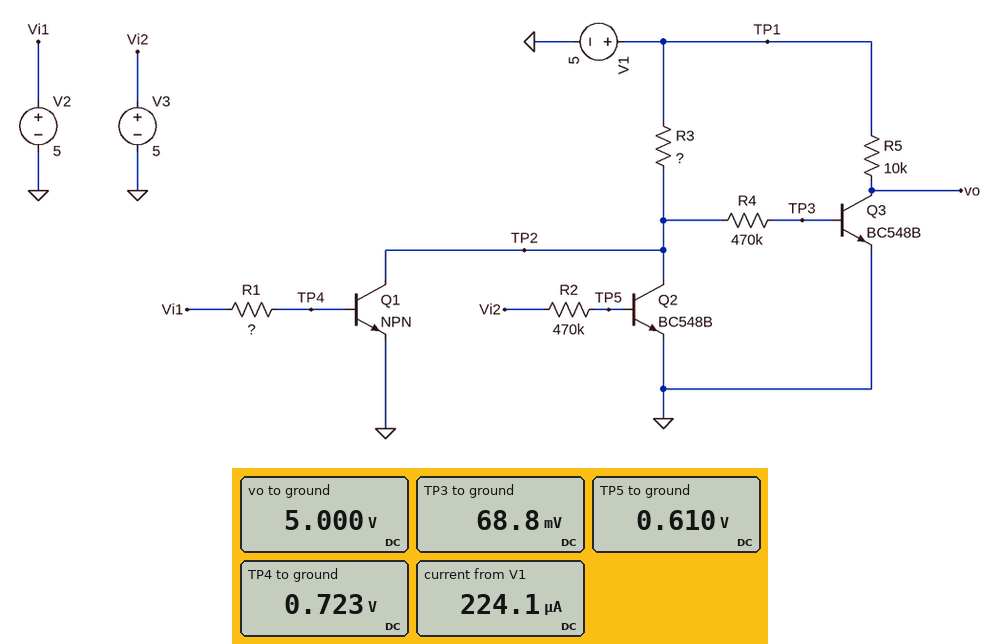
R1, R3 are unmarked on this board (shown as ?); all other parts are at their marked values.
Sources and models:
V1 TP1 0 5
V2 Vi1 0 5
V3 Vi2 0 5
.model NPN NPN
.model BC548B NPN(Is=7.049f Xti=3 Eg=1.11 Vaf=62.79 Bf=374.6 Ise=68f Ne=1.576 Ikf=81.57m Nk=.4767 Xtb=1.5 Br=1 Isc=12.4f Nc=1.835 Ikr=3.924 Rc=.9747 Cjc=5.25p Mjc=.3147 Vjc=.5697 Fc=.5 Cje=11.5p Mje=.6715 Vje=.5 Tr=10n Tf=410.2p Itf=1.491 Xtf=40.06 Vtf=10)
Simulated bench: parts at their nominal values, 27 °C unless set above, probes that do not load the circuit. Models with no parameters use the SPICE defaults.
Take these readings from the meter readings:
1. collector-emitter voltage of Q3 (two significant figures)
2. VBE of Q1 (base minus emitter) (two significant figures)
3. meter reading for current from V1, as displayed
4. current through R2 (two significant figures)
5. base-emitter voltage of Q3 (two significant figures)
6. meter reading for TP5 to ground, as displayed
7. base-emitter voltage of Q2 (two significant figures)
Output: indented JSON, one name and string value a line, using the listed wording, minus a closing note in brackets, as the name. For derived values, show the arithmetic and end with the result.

{
  "collector-emitter voltage of Q3": "5 V = 5.0 V",
  "VBE of Q1 (base minus emitter)": "723 mV = 720 mV",
  "meter reading for current from V1, as displayed": "224.1 µA",
  "current through R2": "(5 V - 610 mV) / 470 kΩ = 9.3 µA",
  "base-emitter voltage of Q3": "68.8 mV = 69 mV",
  "meter reading for TP5 to ground, as displayed": "0.610 V",
  "base-emitter voltage of Q2": "610 mV = 610 mV"
}
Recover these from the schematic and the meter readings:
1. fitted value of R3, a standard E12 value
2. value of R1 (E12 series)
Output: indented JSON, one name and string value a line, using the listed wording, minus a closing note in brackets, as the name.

{
  "fitted value of R3, a standard E12 value": "22 kΩ",
  "value of R1": "390 kΩ"
}
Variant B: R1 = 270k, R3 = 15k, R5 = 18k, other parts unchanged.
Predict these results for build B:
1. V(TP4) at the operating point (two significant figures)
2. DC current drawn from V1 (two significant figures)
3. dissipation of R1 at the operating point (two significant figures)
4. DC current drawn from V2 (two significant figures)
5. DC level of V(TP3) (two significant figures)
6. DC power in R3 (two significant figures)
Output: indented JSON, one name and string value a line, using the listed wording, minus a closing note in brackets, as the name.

{
  "V(TP4) at the operating point": "740 mV",
  "DC current drawn from V1": "330 µA",
  "dissipation of R1 at the operating point": "67 µW",
  "DC current drawn from V2": "16 µA",
  "DC level of V(TP3)": "73 mV",
  "DC power in R3": "1.6 mW"
}
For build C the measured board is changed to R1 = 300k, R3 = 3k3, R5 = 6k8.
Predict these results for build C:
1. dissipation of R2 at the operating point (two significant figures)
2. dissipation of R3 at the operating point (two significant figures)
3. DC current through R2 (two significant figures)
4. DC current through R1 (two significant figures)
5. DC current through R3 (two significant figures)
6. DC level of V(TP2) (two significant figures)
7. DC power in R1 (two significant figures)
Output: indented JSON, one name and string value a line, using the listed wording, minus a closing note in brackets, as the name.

{
  "dissipation of R2 at the operating point": "40 µW",
  "dissipation of R3 at the operating point": "7.2 mW",
  "DC current through R2": "9.2 µA",
  "DC current through R1": "14 µA",
  "DC current through R3": "1.5 mA",
  "DC level of V(TP2)": "120 mV",
  "DC power in R1": "60 µW"
}
